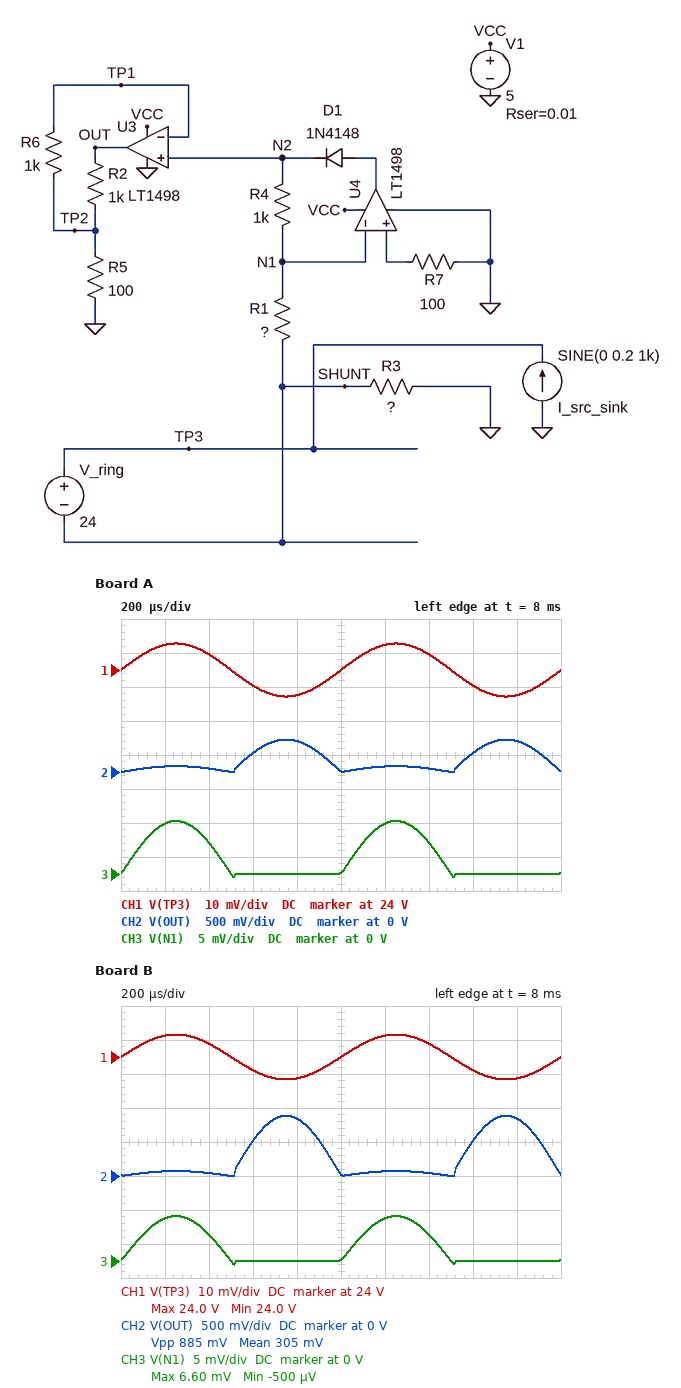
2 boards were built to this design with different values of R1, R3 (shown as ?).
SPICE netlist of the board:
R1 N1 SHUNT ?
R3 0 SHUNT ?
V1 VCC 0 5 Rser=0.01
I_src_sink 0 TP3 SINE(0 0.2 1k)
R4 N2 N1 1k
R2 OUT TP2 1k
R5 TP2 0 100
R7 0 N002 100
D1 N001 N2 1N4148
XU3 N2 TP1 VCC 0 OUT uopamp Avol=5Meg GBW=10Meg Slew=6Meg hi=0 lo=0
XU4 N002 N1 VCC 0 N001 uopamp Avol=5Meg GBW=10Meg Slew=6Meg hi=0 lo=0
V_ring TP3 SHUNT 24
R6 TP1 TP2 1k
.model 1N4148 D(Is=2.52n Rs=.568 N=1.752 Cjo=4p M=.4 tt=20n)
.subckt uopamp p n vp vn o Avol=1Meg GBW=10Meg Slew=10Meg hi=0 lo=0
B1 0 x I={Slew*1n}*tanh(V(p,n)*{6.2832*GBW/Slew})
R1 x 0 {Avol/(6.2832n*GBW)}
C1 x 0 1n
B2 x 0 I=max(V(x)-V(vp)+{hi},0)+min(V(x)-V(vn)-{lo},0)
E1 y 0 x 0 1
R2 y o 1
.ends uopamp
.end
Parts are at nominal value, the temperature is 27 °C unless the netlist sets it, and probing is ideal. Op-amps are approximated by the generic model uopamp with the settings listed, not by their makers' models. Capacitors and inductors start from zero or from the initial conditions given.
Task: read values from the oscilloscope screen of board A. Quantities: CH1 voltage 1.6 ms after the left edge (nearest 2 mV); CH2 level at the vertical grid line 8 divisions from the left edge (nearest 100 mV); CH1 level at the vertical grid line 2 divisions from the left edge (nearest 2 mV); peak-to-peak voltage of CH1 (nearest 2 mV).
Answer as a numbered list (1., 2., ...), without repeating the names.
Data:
1. 23.996 V
2. 300 mV
3. 24.004 V
4. 16 mV
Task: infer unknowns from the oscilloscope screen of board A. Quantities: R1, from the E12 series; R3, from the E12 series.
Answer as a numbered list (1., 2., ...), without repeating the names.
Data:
1. 180 Ω
2. 0.039 Ω
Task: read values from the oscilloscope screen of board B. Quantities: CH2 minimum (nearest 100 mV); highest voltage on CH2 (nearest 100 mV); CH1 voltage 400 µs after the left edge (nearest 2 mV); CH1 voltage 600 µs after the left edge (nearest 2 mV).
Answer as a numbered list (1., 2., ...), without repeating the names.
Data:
1. 0 V
2. 900 mV
3. 24.004 V
4. 23.996 V
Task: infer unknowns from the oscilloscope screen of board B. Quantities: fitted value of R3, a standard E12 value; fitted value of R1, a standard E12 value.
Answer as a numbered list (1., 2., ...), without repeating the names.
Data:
1. 0.033 Ω
2. 82 Ω
